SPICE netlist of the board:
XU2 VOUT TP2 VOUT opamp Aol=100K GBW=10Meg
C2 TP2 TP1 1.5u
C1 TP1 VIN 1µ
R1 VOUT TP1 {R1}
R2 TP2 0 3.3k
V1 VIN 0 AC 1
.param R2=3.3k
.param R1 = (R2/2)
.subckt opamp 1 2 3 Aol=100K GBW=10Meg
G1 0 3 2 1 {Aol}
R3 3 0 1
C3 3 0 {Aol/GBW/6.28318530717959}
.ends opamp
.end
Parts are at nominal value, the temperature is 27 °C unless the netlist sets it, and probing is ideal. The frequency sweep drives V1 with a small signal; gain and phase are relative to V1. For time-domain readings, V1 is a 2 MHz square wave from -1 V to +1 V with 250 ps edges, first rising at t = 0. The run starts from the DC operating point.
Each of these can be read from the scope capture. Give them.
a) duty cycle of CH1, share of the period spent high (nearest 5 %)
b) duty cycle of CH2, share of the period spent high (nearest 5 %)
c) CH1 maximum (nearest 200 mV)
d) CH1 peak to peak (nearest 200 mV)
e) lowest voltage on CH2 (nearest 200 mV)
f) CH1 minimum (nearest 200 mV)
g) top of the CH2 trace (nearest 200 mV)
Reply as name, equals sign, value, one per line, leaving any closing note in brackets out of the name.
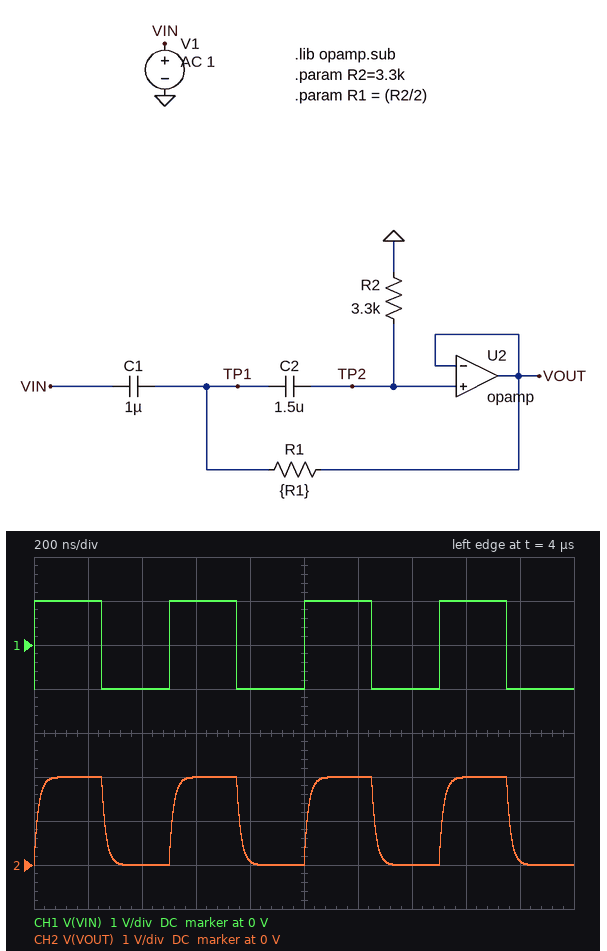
duty cycle of CH1, share of the period spent high = 50 %
duty cycle of CH2, share of the period spent high = 50 %
CH1 maximum = 1.0 V
CH1 peak to peak = 2.0 V
lowest voltage on CH2 = 0 V
CH1 minimum = -1.0 V
top of the CH2 trace = 2.0 V
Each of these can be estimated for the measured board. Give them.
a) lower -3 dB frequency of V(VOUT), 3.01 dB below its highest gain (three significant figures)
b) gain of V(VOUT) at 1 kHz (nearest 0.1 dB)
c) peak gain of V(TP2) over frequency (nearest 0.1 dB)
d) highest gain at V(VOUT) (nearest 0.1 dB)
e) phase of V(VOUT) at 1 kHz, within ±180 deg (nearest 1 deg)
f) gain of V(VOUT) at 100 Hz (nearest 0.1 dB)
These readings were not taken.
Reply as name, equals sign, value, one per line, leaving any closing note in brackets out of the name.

lower -3 dB frequency of V(VOUT), 3.01 dB below its highest gain = 56.9 Hz
gain of V(VOUT) at 1 kHz = 0 dB
peak gain of V(TP2) over frequency = 0 dB
highest gain at V(VOUT) = 0 dB
phase of V(VOUT) at 1 kHz, within ±180 deg = 5 deg
gain of V(VOUT) at 100 Hz = -0.5 dB
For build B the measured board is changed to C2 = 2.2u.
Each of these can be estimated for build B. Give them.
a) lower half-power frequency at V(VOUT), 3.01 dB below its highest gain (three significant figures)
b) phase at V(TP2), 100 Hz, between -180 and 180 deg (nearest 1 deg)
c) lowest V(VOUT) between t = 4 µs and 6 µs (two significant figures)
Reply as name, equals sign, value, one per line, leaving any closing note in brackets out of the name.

lower half-power frequency at V(VOUT), 3.01 dB below its highest gain = 49.9 Hz
phase at V(TP2), 100 Hz, between -180 and 180 deg = 42 deg
lowest V(VOUT) between t = 4 µs and 6 µs = -2.6 mV
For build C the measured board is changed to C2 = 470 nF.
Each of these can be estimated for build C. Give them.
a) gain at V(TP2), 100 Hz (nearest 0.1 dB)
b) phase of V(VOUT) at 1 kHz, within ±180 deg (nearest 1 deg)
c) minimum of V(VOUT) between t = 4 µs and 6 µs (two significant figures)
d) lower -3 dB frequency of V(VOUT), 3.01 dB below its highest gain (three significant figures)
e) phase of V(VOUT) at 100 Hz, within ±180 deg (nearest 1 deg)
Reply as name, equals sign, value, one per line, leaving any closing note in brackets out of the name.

gain at V(TP2), 100 Hz = -3.6 dB
phase of V(VOUT) at 1 kHz, within ±180 deg = 9 deg
minimum of V(VOUT) between t = 4 µs and 6 µs = -5.7 mV
lower -3 dB frequency of V(VOUT), 3.01 dB below its highest gain = 107 Hz
phase of V(VOUT) at 100 Hz, within ±180 deg = 90 deg
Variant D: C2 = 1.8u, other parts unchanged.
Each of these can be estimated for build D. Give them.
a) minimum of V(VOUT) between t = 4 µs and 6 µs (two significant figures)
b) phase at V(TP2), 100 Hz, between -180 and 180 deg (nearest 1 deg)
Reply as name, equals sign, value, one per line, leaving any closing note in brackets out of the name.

minimum of V(VOUT) between t = 4 µs and 6 µs = -2.8 mV
phase at V(TP2), 100 Hz, between -180 and 180 deg = 45 deg
